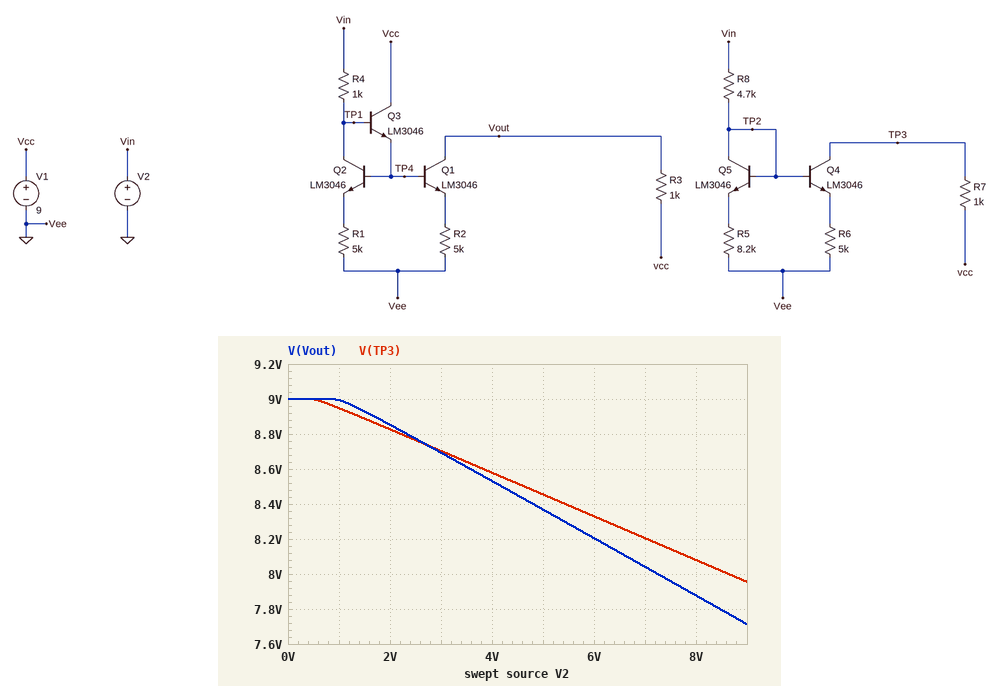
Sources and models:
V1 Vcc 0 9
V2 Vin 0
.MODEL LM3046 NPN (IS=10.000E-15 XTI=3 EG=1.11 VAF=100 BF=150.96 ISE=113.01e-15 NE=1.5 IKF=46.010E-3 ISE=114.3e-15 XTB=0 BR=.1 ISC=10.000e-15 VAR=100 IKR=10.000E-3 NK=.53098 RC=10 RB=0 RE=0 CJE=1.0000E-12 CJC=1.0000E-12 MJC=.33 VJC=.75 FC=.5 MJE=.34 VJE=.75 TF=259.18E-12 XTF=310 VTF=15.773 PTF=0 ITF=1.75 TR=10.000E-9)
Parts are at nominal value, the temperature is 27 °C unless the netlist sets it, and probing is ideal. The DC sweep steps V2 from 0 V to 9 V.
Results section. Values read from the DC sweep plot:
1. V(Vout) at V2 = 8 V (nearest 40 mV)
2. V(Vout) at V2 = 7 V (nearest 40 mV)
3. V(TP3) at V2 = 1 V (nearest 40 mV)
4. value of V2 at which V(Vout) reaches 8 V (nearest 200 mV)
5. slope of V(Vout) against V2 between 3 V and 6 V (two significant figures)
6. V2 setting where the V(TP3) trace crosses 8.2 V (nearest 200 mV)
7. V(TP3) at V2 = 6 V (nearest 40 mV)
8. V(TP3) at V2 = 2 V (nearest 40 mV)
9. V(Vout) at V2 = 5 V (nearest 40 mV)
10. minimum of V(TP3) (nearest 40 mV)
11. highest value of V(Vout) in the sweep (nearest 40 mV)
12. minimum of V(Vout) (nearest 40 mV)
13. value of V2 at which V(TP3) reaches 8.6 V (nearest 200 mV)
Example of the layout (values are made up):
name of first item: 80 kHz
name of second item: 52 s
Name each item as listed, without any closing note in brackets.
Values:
V(Vout) at V2 = 8 V: 7.88 V
V(Vout) at V2 = 7 V: 8.04 V
V(TP3) at V2 = 1 V: 8.96 V
value of V2 at which V(Vout) reaches 8 V: 7.2 V
slope of V(Vout) against V2 between 3 V and 6 V: -0.16 V/V
V2 setting where the V(TP3) trace crosses 8.2 V: 7.0 V
V(TP3) at V2 = 6 V: 8.32 V
V(TP3) at V2 = 2 V: 8.84 V
V(Vout) at V2 = 5 V: 8.36 V
minimum of V(TP3): 7.96 V
highest value of V(Vout) in the sweep: 9.00 V
minimum of V(Vout): 7.72 V
value of V2 at which V(TP3) reaches 8.6 V: 3.8 V
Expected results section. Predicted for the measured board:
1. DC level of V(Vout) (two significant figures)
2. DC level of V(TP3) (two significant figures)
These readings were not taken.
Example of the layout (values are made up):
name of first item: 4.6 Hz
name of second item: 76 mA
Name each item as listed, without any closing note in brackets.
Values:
DC level of V(Vout): 9.0 V
DC level of V(TP3): 9.0 V
